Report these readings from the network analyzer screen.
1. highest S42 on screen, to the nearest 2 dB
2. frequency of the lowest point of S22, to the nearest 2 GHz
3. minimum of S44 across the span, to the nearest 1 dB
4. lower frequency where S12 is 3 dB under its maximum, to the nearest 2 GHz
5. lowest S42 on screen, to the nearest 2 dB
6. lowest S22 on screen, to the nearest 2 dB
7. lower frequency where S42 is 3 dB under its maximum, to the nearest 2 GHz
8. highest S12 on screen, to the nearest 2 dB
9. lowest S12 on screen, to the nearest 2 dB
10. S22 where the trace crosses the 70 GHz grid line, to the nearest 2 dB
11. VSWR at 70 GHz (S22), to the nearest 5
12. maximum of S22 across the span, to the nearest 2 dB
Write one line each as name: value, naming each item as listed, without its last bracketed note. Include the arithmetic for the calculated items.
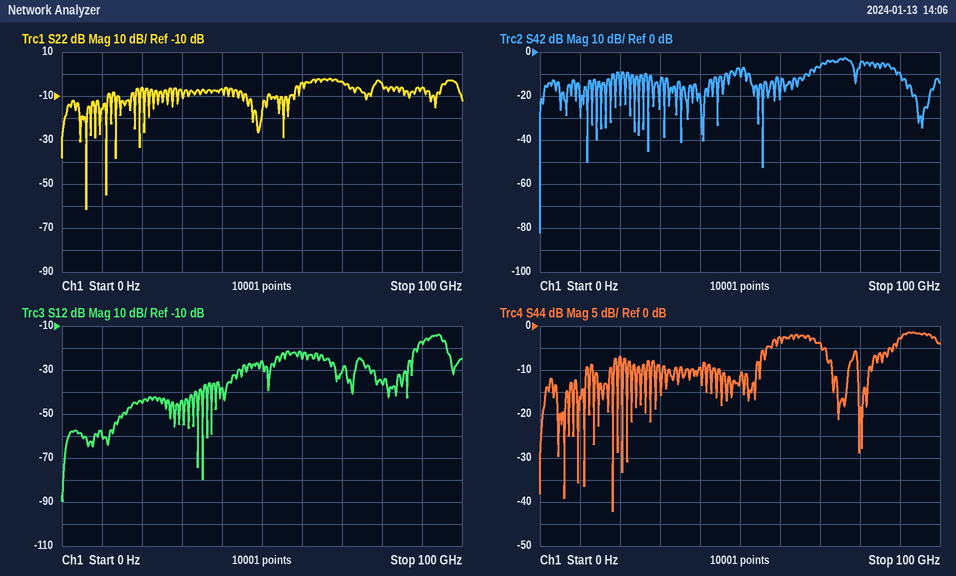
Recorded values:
highest S42 on screen, to the nearest 2 dB: -2 dB
frequency of the lowest point of S22, to the nearest 2 GHz: 6 GHz
minimum of S44 across the span, to the nearest 1 dB: -42 dB
lower frequency where S12 is 3 dB under its maximum, to the nearest 2 GHz: 90 GHz
lowest S42 on screen, to the nearest 2 dB: -82 dB
lowest S22 on screen, to the nearest 2 dB: -62 dB
lower frequency where S42 is 3 dB under its maximum, to the nearest 2 GHz: 70 GHz
highest S12 on screen, to the nearest 2 dB: -14 dB
lowest S12 on screen, to the nearest 2 dB: -90 dB
S22 where the trace crosses the 70 GHz grid line, to the nearest 2 dB: -4 dB
VSWR at 70 GHz (S22), to the nearest 5: |Γ| = 10^(-4/20) = 0.6310; VSWR = (1 + 0.6310)/(1 − 0.6310) ≈ 4.42, so 5 to the nearest 5
maximum of S22 across the span, to the nearest 2 dB: -2 dB
